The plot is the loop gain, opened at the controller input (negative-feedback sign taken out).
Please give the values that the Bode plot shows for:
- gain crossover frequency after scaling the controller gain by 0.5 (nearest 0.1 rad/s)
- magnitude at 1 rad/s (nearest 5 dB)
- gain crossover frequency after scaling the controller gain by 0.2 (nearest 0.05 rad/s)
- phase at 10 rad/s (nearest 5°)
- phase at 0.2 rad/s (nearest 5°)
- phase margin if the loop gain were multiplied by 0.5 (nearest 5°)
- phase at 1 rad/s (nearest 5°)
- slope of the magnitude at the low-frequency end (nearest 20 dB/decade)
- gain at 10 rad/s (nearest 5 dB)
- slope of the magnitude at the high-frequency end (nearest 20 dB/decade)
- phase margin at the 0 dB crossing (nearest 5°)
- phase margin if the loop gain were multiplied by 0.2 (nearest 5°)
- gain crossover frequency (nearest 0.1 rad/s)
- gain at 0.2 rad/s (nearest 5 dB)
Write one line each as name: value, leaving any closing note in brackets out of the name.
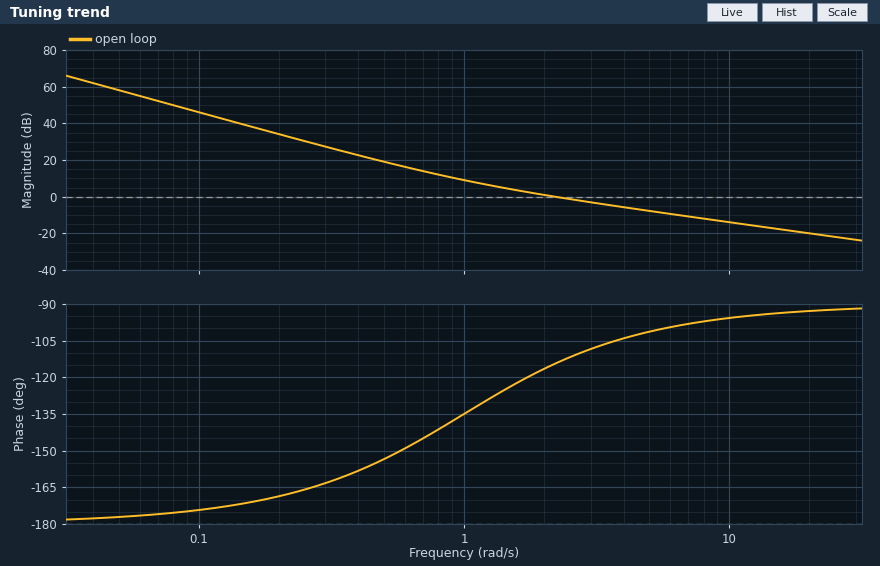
gain crossover frequency after scaling the controller gain by 0.5: 1.3 rad/s
magnitude at 1 rad/s: 10 dB
gain crossover frequency after scaling the controller gain by 0.2: 0.70 rad/s
phase at 10 rad/s: -95°
phase at 0.2 rad/s: -170°
phase margin if the loop gain were multiplied by 0.5: 50°
phase at 1 rad/s: -135°
slope of the magnitude at the low-frequency end: -40 dB/decade
gain at 10 rad/s: -15 dB
slope of the magnitude at the high-frequency end: -20 dB/decade
phase margin at the 0 dB crossing: 65°
phase margin if the loop gain were multiplied by 0.2: 35°
gain crossover frequency: 2.2 rad/s
gain at 0.2 rad/s: 35 dB
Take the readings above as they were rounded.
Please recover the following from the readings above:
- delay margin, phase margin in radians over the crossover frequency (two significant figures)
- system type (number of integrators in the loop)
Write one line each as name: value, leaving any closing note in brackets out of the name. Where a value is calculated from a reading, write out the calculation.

delay margin, phase margin in radians over the crossover frequency: 65 × π / 180 / 2.2 = 0.52 s
system type: 2
